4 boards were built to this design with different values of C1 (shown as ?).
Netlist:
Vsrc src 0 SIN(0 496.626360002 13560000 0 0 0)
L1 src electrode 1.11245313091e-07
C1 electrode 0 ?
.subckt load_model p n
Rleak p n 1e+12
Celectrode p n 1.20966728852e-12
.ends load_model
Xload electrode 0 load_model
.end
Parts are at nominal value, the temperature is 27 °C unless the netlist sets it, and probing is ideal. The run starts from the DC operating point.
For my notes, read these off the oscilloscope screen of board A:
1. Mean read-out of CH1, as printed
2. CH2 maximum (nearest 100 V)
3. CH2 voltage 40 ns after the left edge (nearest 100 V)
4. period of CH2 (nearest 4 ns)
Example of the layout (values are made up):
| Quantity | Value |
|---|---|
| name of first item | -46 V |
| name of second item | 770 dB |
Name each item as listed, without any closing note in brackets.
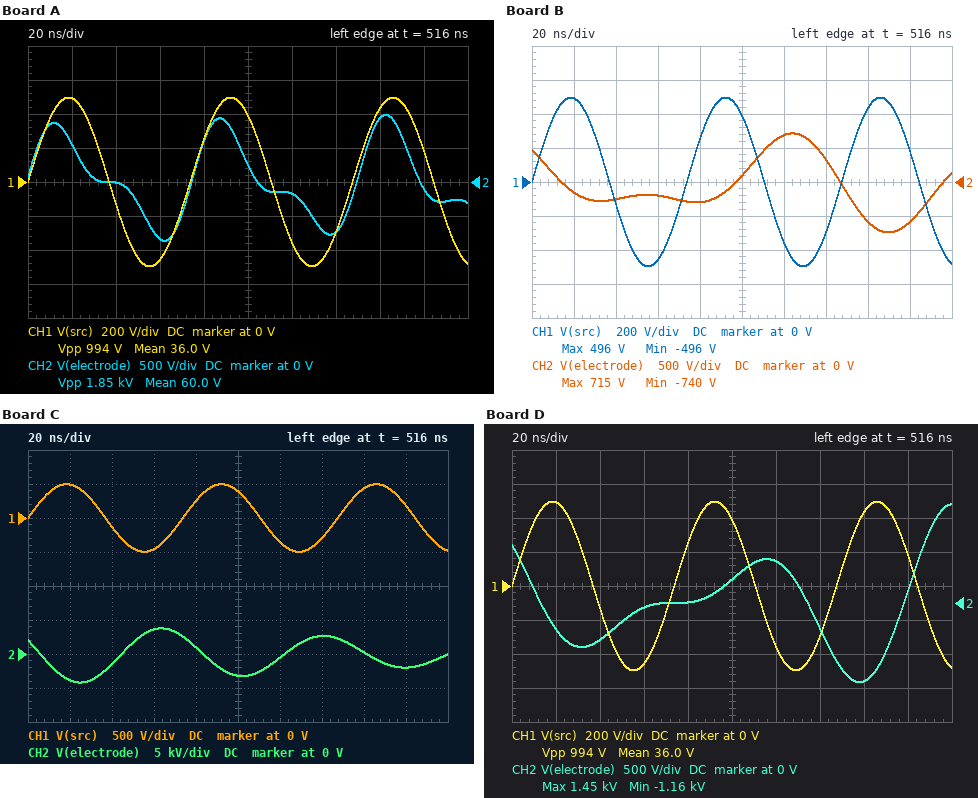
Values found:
| Quantity | Value |
|---|---|
| Mean read-out of CH1, as printed | 36.0 V |
| CH2 maximum | 1.0 kV |
| CH2 voltage 40 ns after the left edge | 0 V |
| period of CH2 | 76 ns |
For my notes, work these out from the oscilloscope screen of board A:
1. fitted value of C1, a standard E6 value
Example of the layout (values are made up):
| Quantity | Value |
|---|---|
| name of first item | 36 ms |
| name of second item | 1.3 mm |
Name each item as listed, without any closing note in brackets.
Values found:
| Quantity | Value |
|---|---|
| fitted value of C1, a standard E6 value | 330 pF |
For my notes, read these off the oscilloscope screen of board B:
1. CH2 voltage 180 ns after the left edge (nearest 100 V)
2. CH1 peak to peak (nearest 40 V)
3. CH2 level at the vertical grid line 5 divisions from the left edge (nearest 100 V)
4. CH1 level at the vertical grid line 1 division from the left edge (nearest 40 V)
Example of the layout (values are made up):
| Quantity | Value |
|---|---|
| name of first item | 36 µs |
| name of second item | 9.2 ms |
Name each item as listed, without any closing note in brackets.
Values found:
| Quantity | Value |
|---|---|
| CH2 voltage 180 ns after the left edge | -600 V |
| CH1 peak to peak | 1.00 kV |
| CH2 level at the vertical grid line 5 divisions from the left edge | 100 V |
| CH1 level at the vertical grid line 1 division from the left edge | 480 V |
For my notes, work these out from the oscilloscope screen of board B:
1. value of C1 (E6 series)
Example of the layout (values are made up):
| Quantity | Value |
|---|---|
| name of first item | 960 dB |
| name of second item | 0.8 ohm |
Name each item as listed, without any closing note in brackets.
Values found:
| Quantity | Value |
|---|---|
| value of C1 | 3.3 nF |
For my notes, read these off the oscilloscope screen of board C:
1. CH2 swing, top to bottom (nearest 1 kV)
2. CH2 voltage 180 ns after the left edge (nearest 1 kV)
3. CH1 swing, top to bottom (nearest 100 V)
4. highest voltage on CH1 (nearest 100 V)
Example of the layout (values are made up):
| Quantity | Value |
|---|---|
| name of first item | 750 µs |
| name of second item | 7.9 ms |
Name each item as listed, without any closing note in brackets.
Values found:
| Quantity | Value |
|---|---|
| CH2 swing, top to bottom | 8 kV |
| CH2 voltage 180 ns after the left edge | -2 kV |
| CH1 swing, top to bottom | 1.0 kV |
| highest voltage on CH1 | 500 V |
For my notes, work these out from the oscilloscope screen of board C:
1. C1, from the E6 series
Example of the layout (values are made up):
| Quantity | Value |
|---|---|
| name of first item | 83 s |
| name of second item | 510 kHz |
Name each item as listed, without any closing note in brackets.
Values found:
| Quantity | Value |
|---|---|
| C1, from the E6 series | 1.5 nF |
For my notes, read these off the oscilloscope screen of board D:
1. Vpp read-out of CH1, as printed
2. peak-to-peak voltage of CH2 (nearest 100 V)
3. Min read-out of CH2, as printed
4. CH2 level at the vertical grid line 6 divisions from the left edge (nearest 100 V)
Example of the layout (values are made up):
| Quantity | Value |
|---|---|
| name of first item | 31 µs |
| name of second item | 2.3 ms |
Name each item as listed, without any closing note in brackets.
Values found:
| Quantity | Value |
|---|---|
| Vpp read-out of CH1, as printed | 994 V |
| peak-to-peak voltage of CH2 | 2.6 kV |
| Min read-out of CH2, as printed | -1.16 kV |
| CH2 level at the vertical grid line 6 divisions from the left edge | 600 V |
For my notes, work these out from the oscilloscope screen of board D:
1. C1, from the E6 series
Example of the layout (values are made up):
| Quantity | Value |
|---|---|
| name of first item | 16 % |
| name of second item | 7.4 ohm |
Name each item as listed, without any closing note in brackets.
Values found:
| Quantity | Value |
|---|---|
| C1, from the E6 series | 2.2 nF |
